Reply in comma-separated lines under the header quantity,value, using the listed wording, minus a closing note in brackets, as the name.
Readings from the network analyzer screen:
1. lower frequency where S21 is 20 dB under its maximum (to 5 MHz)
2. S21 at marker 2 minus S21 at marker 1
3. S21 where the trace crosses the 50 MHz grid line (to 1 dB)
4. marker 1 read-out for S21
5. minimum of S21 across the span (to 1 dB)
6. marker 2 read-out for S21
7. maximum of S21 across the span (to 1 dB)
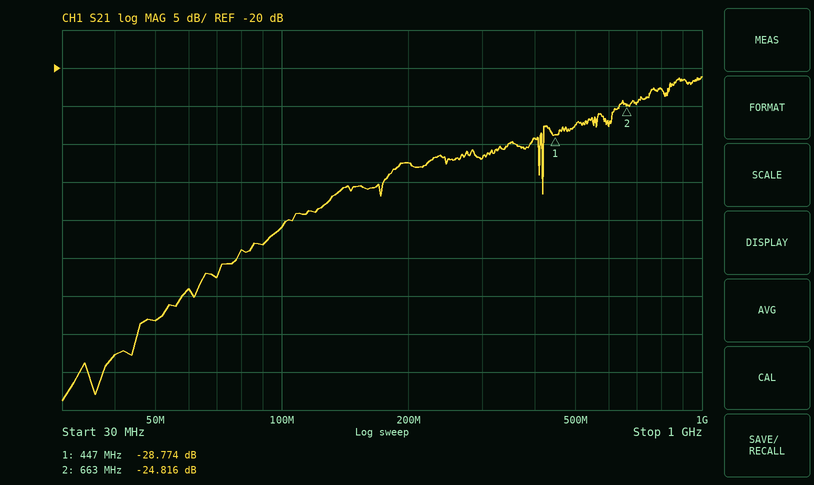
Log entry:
quantity,value
lower frequency where S21 is 20 dB under its maximum,100 MHz
S21 at marker 2 minus S21 at marker 1,3.958 dB
S21 where the trace crosses the 50 MHz grid line,-53 dB
marker 1 read-out for S21,-28.774 dB
minimum of S21 across the span,-64 dB
marker 2 read-out for S21,-24.816 dB
maximum of S21 across the span,-21 dB
